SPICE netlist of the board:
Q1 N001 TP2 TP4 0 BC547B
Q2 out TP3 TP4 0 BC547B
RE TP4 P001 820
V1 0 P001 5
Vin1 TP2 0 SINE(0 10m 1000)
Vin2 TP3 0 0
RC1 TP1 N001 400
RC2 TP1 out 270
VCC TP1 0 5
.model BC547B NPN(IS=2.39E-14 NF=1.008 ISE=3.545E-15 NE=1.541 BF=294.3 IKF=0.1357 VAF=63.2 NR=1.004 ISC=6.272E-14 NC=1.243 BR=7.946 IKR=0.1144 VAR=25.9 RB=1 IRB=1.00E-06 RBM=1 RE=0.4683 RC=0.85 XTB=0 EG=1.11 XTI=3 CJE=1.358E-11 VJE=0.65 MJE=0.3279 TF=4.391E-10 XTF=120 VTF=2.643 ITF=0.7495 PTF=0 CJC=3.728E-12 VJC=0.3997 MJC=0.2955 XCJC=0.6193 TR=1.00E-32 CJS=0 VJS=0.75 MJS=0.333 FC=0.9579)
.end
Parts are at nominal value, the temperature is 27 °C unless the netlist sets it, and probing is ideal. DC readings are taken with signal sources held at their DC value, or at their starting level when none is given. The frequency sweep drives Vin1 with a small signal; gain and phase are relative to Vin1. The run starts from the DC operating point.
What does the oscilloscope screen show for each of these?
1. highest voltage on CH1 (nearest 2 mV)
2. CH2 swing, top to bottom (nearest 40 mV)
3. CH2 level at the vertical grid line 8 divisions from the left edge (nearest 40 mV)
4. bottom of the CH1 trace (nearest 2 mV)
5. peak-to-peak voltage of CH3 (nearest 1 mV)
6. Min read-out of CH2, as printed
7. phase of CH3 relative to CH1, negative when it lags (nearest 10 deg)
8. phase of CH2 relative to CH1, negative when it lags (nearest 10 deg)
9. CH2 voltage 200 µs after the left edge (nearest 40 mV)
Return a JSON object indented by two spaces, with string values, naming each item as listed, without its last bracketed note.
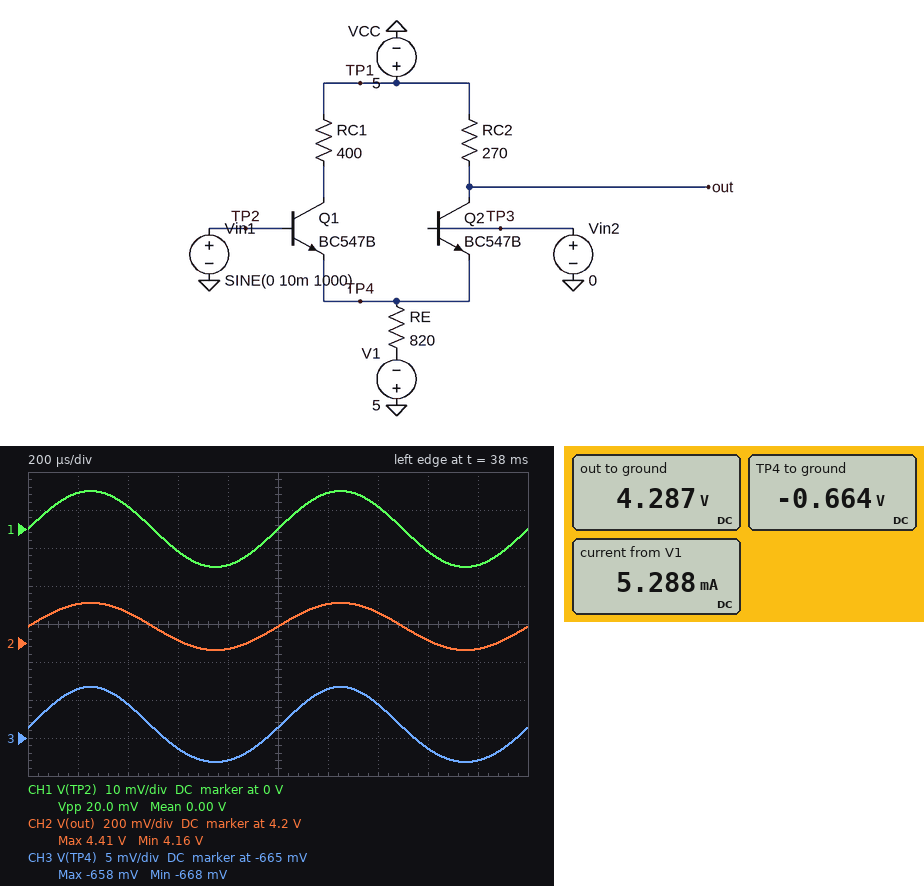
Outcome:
{
  "highest voltage on CH1": "10 mV",
  "CH2 swing, top to bottom": "240 mV",
  "CH2 level at the vertical grid line 8 divisions from the left edge": "4.20 V",
  "bottom of the CH1 trace": "-10 mV",
  "peak-to-peak voltage of CH3": "10 mV",
  "Min read-out of CH2, as printed": "4.16 V",
  "phase of CH3 relative to CH1, negative when it lags": "0 deg",
  "phase of CH2 relative to CH1, negative when it lags": "0 deg",
  "CH2 voltage 200 µs after the left edge": "4.40 V"
}
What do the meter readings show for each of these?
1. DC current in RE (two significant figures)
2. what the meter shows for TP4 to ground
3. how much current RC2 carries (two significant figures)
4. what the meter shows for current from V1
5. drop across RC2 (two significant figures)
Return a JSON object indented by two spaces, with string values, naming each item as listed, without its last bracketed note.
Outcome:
{
  "DC current in RE": "5.3 mA",
  "what the meter shows for TP4 to ground": "-0.664 V",
  "how much current RC2 carries": "2.6 mA",
  "what the meter shows for current from V1": "5.288 mA",
  "drop across RC2": "710 mV"
}
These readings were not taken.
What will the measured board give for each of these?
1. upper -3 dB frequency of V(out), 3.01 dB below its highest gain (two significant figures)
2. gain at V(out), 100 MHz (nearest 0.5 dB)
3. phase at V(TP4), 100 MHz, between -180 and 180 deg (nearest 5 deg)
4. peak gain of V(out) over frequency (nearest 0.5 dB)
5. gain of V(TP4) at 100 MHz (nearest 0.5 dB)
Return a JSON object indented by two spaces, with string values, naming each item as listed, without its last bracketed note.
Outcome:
{
  "upper -3 dB frequency of V(out), 3.01 dB below its highest gain": "290 MHz",
  "gain at V(out), 100 MHz": "21.5 dB",
  "phase at V(TP4), 100 MHz, between -180 and 180 deg": "0 deg",
  "peak gain of V(out) over frequency": "22.0 dB",
  "gain of V(TP4) at 100 MHz": "-6.0 dB"
}
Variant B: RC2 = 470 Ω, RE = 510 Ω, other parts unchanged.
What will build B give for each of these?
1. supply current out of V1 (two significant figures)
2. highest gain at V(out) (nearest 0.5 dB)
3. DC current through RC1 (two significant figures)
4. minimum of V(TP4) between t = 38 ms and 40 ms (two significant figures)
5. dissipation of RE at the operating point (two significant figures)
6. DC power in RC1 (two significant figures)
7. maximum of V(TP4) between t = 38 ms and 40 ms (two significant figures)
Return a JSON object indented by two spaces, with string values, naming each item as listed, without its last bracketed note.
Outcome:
{
  "supply current out of V1": "8.5 mA",
  "highest gain at V(out)": "30.5 dB",
  "DC current through RC1": "4.2 mA",
  "minimum of V(TP4) between t = 38 ms and 40 ms": "-680 mV",
  "dissipation of RE at the operating point": "37 mW",
  "DC power in RC1": "7.2 mW",
  "maximum of V(TP4) between t = 38 ms and 40 ms": "-670 mV"
}
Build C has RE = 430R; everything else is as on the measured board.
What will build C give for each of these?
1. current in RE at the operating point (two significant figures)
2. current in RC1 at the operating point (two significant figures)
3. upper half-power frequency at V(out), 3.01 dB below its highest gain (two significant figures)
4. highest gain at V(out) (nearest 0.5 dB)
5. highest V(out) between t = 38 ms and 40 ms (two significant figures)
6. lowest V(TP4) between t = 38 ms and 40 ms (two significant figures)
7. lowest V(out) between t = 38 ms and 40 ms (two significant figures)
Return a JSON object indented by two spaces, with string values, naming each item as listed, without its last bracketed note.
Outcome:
{
  "current in RE at the operating point": "10 mA",
  "current in RC1 at the operating point": "5.0 mA",
  "upper half-power frequency at V(out), 3.01 dB below its highest gain": "250 MHz",
  "highest gain at V(out)": "27.0 dB",
  "highest V(out) between t = 38 ms and 40 ms": "3.9 V",
  "lowest V(TP4) between t = 38 ms and 40 ms": "-690 mV",
  "lowest V(out) between t = 38 ms and 40 ms": "3.4 V"
}
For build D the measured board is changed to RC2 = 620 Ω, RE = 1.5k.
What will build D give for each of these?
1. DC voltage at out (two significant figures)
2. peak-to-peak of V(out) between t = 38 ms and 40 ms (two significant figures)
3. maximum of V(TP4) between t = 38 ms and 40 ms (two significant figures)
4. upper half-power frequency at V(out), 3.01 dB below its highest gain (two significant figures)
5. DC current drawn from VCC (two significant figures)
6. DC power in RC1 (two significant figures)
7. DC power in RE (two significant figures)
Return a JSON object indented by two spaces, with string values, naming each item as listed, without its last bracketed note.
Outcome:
{
  "DC voltage at out": "4.1 V",
  "peak-to-peak of V(out) between t = 38 ms and 40 ms": "320 mV",
  "maximum of V(TP4) between t = 38 ms and 40 ms": "-640 mV",
  "upper half-power frequency at V(out), 3.01 dB below its highest gain": "140 MHz",
  "DC current drawn from VCC": "2.9 mA",
  "DC power in RC1": "840 µW",
  "DC power in RE": "13 mW"
}
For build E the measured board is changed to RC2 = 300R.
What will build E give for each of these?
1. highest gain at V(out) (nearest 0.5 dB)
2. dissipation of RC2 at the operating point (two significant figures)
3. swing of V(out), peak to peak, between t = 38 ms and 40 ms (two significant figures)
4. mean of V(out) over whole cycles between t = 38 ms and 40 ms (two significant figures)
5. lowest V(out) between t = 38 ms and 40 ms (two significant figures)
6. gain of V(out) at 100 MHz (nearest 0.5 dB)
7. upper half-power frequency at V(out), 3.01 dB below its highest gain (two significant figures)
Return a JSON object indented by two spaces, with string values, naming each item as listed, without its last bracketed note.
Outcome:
{
  "highest gain at V(out)": "23.0 dB",
  "dissipation of RC2 at the operating point": "2.1 mW",
  "swing of V(out), peak to peak, between t = 38 ms and 40 ms": "280 mV",
  "mean of V(out) over whole cycles between t = 38 ms and 40 ms": "4.2 V",
  "lowest V(out) between t = 38 ms and 40 ms": "4.1 V",
  "gain of V(out) at 100 MHz": "22.5 dB",
  "upper half-power frequency at V(out), 3.01 dB below its highest gain": "260 MHz"
}
